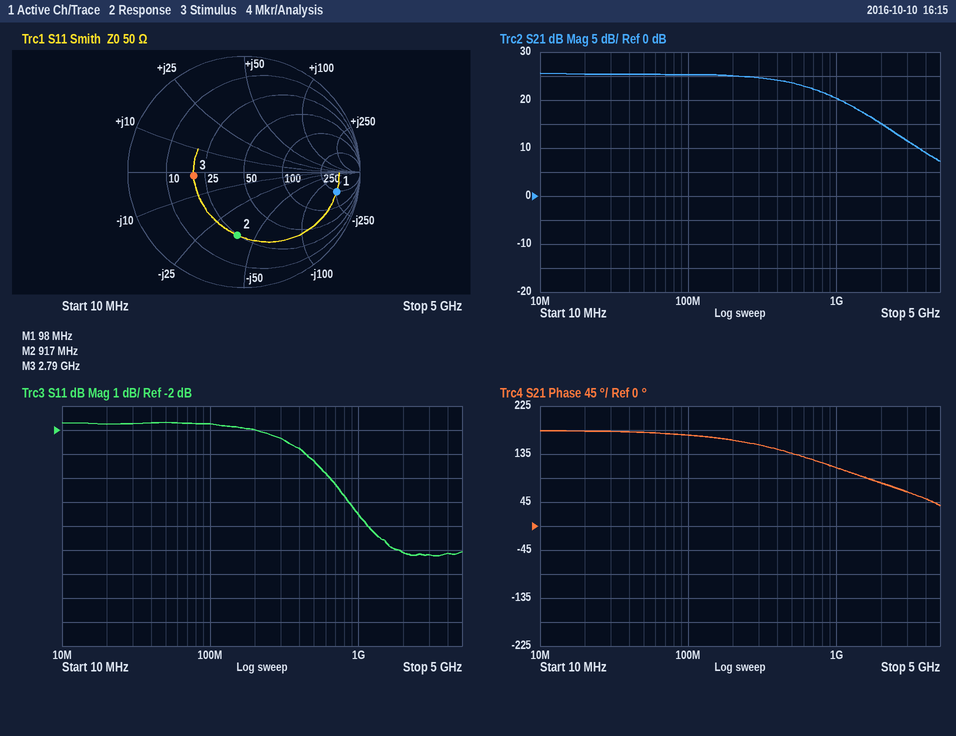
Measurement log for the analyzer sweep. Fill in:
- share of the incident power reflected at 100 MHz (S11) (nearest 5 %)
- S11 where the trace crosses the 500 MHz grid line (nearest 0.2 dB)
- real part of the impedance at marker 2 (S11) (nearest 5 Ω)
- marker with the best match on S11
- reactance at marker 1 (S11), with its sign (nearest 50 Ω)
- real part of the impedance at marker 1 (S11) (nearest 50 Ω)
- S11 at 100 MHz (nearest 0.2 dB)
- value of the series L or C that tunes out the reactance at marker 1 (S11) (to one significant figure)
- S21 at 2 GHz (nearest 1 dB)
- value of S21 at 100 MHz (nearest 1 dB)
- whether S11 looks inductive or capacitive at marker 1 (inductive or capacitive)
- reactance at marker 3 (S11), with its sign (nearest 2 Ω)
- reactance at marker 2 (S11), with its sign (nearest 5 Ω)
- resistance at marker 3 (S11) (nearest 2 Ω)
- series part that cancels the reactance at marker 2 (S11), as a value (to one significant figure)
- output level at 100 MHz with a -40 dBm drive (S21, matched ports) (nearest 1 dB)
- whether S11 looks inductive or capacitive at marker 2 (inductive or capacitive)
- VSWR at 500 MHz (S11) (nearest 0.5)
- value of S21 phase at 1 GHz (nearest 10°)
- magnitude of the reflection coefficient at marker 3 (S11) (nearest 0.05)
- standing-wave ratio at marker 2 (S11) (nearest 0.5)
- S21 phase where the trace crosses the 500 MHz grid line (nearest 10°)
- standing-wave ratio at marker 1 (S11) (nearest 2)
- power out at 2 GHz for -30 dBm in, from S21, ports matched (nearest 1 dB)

65 %
-3.2 dB
25 Ω
marker 3
-250 Ω
250 Ω
-1.8 dB
400 nH
15 dB
25 dB
capacitive
-2 Ω
-40 Ω
20 Ω
7 nH
-15 dBm
capacitive
5.5
110°
0.45
3.5
140°
10
-15 dBm
